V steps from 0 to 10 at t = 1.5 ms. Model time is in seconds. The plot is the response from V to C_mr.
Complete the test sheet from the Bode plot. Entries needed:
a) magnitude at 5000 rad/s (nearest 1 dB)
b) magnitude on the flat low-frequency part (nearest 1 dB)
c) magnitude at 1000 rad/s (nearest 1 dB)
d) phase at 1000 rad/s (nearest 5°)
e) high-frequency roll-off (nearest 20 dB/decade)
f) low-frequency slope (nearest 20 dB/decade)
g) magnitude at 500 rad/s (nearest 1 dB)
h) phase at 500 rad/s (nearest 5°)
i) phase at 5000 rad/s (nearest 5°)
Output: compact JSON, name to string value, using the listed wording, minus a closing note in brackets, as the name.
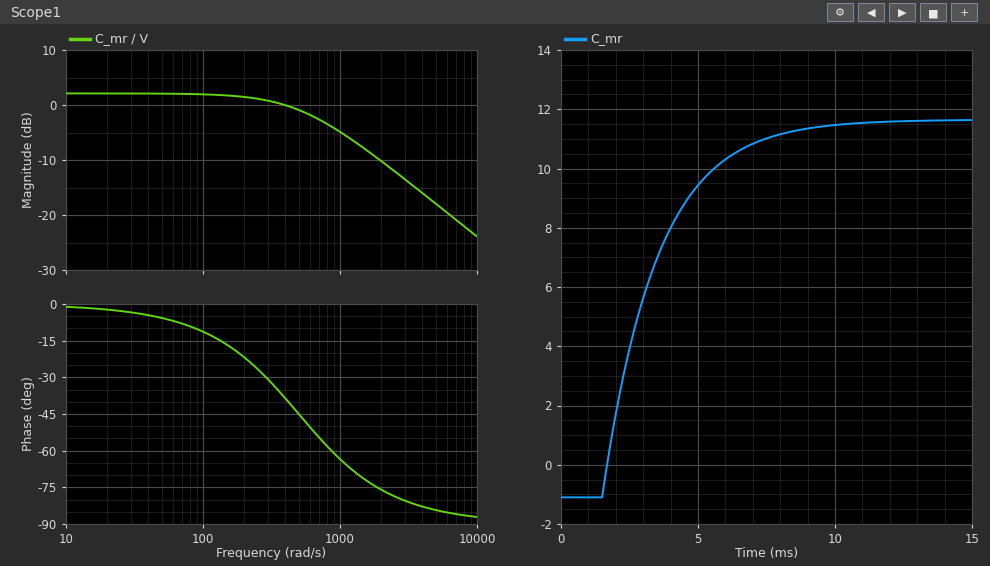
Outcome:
{"magnitude at 5000 rad/s": "-18 dB", "magnitude on the flat low-frequency part": "2 dB", "magnitude at 1000 rad/s": "-5 dB", "phase at 1000 rad/s": "-65°", "high-frequency roll-off": "-20 dB/decade", "low-frequency slope": "0 dB/decade", "magnitude at 500 rad/s": "-1 dB", "phase at 500 rad/s": "-45°", "phase at 5000 rad/s": "-85°"}
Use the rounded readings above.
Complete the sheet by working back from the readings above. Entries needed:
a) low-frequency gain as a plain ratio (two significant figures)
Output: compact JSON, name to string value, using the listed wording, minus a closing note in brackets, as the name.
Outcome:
{"low-frequency gain as a plain ratio": "1.3"}
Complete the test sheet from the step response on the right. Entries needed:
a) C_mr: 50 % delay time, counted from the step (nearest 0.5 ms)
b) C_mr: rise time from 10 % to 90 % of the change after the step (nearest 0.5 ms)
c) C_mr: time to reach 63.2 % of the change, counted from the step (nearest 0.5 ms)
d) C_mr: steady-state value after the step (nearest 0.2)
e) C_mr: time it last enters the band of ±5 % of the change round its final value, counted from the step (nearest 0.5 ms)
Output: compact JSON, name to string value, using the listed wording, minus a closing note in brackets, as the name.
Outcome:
{"C_mr: 50 % delay time, counted from the step": "1.5 ms", "C_mr: rise time from 10 % to 90 % of the change after the step": "4.5 ms", "C_mr: time to reach 63.2 % of the change, counted from the step": "2.0 ms", "C_mr: steady-state value after the step": "11.6", "C_mr: time it last enters the band of ±5 % of the change round its final value, counted from the step": "6.0 ms"}
